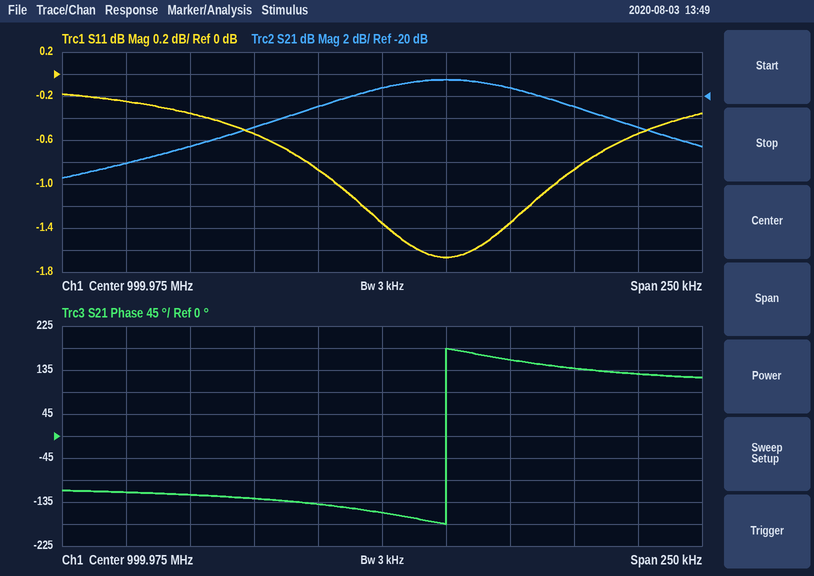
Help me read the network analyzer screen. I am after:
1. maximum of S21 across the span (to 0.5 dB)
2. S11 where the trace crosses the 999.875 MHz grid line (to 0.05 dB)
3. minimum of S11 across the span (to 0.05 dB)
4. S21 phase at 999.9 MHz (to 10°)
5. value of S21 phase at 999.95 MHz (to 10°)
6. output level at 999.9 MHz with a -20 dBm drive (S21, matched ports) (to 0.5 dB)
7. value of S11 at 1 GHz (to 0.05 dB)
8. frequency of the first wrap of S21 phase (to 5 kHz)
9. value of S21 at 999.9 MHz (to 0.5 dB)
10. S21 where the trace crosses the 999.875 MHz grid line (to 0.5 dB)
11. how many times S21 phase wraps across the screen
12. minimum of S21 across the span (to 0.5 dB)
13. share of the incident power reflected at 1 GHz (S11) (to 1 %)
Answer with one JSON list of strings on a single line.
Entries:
["-18.5 dB", "-0.25 dB", "-1.65 dB", "-120°", "-140°", "-44.5 dBm", "-1.65 dB", "1.000000 GHz", "-24.5 dB", "-26.0 dB", "1", "-27.5 dB", "68 %"]
